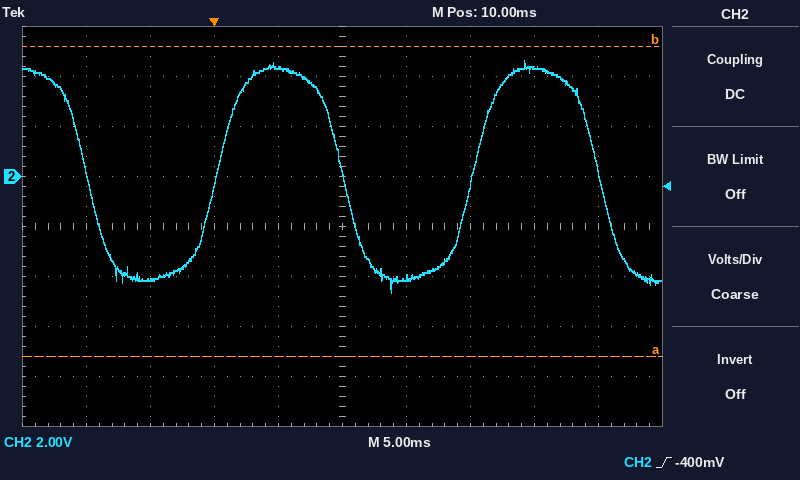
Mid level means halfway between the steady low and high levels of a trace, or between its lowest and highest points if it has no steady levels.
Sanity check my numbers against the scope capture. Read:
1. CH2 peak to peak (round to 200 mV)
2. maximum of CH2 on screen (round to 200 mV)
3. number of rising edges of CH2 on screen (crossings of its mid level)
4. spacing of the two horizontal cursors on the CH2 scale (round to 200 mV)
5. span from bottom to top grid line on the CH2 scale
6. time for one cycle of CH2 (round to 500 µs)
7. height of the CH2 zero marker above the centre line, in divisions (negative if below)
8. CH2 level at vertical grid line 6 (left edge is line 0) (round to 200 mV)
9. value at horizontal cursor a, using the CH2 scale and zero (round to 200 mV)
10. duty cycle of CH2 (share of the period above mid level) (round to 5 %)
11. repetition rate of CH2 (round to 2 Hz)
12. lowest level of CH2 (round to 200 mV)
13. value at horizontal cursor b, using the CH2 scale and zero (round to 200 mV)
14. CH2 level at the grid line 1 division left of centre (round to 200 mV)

9.2 V
4.6 V
2
12.4 V
16 V
20.0 ms
+1.0 div
-4.0 V
-7.2 V
50 %
50 Hz
-4.6 V
5.2 V
4.4 V
